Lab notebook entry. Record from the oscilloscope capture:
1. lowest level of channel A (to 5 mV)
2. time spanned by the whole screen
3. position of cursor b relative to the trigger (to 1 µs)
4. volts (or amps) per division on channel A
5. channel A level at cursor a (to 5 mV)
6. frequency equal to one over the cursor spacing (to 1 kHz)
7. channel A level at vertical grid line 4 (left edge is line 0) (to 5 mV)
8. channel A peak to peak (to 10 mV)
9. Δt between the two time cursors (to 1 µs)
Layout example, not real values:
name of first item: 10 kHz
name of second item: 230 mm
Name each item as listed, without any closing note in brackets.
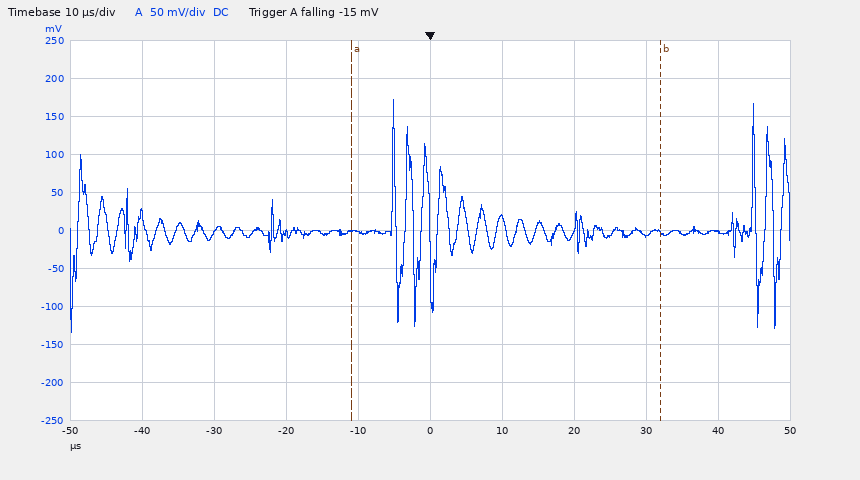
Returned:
lowest level of channel A: -135 mV
time spanned by the whole screen: 100 µs
position of cursor b relative to the trigger: +32 µs
volts (or amps) per division on channel A: 50 mV
channel A level at cursor a: 0 mV
frequency equal to one over the cursor spacing: 23 kHz
channel A level at vertical grid line 4 (left edge is line 0): 0 mV
channel A peak to peak: 310 mV
Δt between the two time cursors: 43 µs
